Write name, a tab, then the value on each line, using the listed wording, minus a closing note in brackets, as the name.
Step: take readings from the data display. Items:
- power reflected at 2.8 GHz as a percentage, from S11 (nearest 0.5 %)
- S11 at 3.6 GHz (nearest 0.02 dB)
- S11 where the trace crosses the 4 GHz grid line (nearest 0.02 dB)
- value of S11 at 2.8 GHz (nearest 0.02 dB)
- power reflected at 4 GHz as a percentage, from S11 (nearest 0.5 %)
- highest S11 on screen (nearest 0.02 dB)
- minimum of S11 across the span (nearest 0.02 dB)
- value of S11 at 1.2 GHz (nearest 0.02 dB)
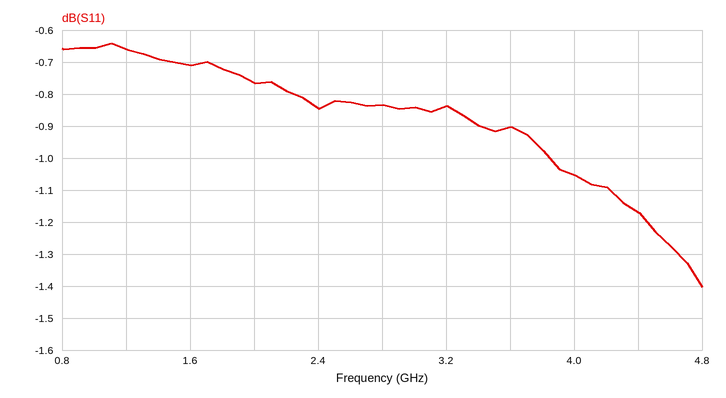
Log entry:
power reflected at 2.8 GHz as a percentage, from S11	82.5 %
S11 at 3.6 GHz	-0.90 dB
S11 where the trace crosses the 4 GHz grid line	-1.06 dB
value of S11 at 2.8 GHz	-0.84 dB
power reflected at 4 GHz as a percentage, from S11	78.5 %
highest S11 on screen	-0.64 dB
minimum of S11 across the span	-1.40 dB
value of S11 at 1.2 GHz	-0.66 dB
